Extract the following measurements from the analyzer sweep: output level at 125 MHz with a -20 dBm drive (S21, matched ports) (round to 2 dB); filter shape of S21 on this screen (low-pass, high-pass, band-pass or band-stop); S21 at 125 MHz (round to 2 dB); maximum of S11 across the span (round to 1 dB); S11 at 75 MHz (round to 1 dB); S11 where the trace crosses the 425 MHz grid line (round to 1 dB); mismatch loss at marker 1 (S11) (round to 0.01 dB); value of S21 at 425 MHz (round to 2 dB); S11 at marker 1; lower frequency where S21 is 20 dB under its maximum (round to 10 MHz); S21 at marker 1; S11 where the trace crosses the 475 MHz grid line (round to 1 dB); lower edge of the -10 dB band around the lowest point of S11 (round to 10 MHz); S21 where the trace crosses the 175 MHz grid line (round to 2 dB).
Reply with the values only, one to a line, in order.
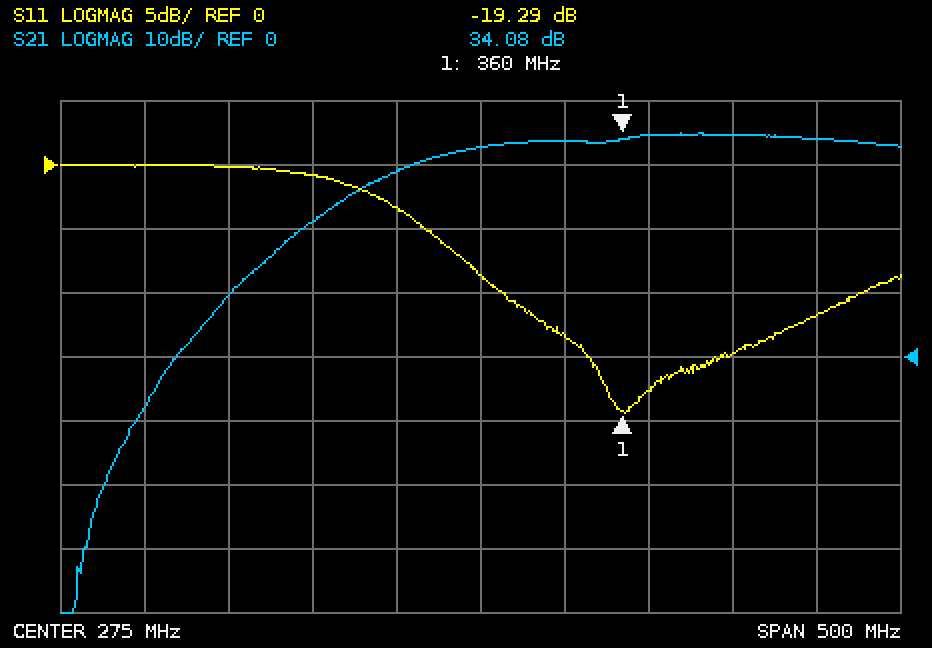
-10 dBm
high-pass
10 dB
0 dB
0 dB
-15 dB
0.05 dB
34 dB
-19.29 dB
150 MHz
34.08 dB
-12 dB
290 MHz
22 dB
